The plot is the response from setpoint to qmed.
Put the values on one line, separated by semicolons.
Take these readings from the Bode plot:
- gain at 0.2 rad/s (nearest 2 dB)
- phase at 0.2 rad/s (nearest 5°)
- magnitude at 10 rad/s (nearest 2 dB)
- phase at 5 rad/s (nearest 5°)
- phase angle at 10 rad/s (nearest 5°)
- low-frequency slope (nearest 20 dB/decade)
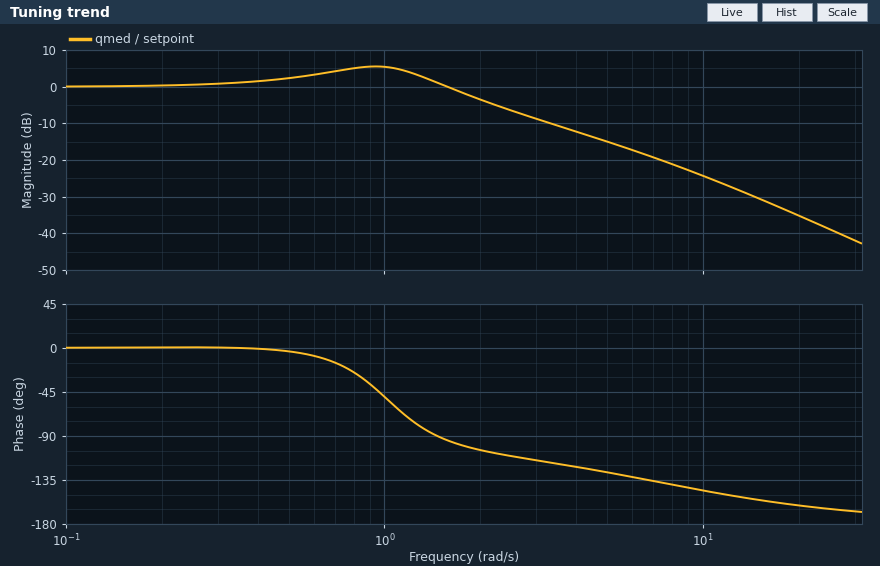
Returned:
0 dB; 0°; -24 dB; -125°; -145°; 0 dB/decade
